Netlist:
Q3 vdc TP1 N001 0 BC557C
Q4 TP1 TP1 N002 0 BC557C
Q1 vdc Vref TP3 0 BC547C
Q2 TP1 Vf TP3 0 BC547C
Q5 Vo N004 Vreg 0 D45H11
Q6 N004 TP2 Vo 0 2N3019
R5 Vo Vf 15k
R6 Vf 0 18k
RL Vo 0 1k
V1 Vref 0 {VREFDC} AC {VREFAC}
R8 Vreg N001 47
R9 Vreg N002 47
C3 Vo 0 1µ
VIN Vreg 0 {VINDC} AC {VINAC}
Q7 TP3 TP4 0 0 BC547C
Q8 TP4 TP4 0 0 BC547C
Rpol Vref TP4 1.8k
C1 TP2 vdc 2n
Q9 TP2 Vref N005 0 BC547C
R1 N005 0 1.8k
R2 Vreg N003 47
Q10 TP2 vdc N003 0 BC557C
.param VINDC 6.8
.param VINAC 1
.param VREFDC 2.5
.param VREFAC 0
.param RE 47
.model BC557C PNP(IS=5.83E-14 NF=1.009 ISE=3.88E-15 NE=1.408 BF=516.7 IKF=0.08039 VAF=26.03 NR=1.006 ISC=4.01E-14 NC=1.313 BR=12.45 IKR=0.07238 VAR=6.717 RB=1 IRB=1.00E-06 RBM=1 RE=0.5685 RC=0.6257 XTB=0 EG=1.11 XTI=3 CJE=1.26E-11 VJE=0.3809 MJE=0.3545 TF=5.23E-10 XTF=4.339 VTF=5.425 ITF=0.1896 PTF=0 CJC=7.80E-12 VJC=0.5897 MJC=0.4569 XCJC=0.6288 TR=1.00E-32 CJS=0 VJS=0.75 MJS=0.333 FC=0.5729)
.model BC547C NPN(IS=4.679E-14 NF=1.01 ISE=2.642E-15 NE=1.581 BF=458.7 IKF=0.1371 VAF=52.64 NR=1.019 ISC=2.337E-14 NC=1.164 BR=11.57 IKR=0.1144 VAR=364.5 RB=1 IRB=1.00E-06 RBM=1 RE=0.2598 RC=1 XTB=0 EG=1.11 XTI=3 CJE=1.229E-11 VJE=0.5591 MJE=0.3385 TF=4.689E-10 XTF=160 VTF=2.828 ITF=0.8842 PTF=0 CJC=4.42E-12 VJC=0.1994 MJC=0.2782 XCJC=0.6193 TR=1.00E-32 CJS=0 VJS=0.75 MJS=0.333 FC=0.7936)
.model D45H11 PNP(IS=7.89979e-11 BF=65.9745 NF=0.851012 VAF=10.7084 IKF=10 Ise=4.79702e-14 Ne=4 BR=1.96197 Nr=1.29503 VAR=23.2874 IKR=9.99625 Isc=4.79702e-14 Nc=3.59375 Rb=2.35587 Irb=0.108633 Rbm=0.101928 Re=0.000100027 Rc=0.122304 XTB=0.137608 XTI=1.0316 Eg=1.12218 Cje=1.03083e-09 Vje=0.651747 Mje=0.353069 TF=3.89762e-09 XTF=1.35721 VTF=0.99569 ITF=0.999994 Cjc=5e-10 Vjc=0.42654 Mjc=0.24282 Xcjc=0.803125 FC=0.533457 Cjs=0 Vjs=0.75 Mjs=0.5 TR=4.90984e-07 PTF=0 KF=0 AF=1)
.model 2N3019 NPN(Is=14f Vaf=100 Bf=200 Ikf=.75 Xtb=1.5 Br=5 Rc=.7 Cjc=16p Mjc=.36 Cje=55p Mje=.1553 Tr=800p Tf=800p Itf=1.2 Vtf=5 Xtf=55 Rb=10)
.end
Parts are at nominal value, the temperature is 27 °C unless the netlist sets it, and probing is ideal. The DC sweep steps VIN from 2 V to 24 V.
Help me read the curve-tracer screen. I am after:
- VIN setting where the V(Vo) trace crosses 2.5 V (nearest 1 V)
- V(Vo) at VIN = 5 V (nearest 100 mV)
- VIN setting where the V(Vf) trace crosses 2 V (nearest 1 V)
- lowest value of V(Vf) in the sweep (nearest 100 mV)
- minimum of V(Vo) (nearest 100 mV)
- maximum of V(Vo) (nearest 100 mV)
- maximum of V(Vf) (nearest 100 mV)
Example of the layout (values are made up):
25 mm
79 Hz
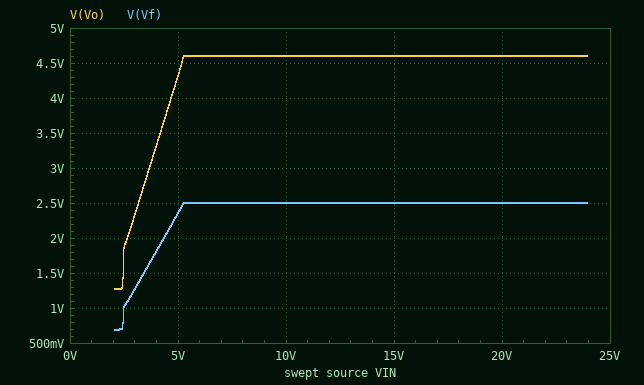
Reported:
3 V
4.3 V
4 V
700 mV
1.3 V
4.6 V
2.5 V
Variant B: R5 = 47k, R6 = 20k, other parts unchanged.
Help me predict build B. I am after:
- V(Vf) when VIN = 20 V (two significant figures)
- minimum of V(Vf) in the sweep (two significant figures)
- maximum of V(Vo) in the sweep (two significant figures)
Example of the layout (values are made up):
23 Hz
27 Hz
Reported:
2.5 V
380 mV
8.4 V
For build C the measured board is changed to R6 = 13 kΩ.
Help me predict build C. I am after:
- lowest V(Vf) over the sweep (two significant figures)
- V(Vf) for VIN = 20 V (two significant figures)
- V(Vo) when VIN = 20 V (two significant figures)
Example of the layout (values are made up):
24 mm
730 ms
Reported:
590 mV
2.5 V
5.4 V
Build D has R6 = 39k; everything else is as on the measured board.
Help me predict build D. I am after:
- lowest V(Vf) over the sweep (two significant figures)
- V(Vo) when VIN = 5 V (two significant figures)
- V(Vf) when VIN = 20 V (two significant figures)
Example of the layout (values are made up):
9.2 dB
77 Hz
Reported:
920 mV
3.5 V
2.5 V
